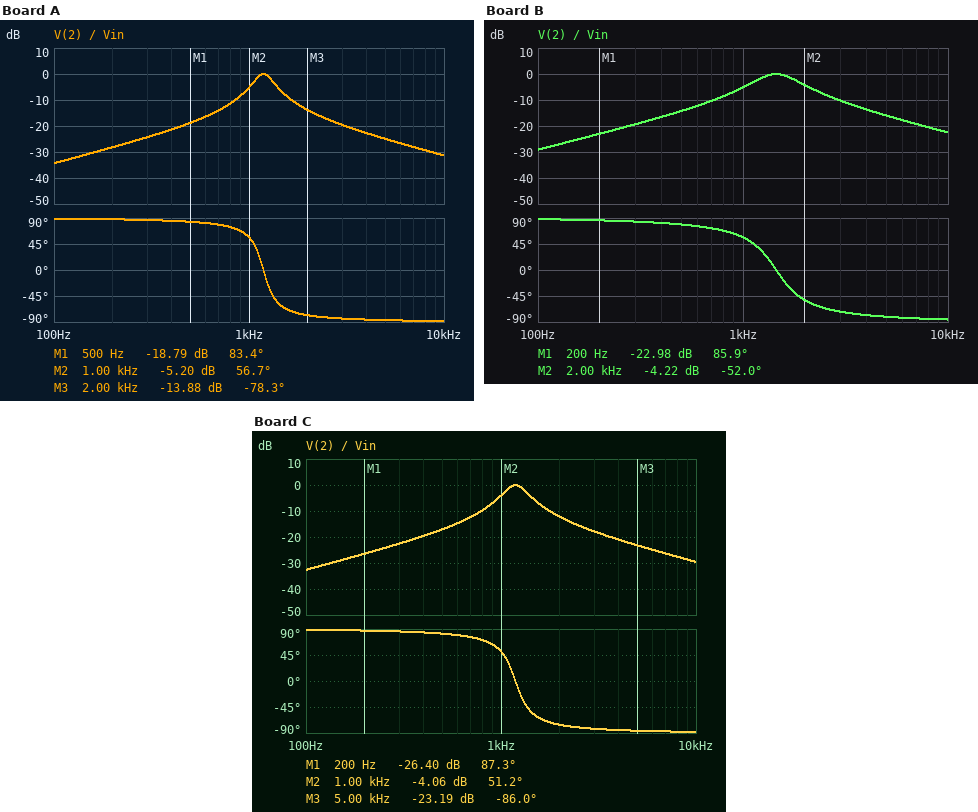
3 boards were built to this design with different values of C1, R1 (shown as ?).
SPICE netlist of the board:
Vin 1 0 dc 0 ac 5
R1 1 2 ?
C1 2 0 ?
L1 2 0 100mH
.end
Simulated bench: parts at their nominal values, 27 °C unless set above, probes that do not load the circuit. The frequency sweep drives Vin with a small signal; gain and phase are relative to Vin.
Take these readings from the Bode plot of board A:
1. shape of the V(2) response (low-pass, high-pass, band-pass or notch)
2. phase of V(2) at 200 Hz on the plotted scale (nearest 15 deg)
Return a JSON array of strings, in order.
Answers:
["band-pass", "90 deg"]
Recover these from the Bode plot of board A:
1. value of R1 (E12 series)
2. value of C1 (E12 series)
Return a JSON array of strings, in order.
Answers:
["3.3 kΩ", "180 nF"]
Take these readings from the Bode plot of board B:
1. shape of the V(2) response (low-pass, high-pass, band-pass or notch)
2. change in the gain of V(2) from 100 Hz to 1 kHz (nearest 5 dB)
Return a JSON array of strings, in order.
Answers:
["band-pass", "25 dB"]
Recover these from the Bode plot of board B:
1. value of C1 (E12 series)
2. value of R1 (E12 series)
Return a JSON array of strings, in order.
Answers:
["120 nF", "1.8 kΩ"]
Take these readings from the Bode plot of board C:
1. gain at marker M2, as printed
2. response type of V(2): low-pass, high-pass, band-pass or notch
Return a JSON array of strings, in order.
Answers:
["-4.06 dB", "band-pass"]
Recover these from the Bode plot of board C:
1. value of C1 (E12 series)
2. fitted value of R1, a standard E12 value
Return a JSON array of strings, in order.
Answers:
["180 nF", "2.7 kΩ"]
